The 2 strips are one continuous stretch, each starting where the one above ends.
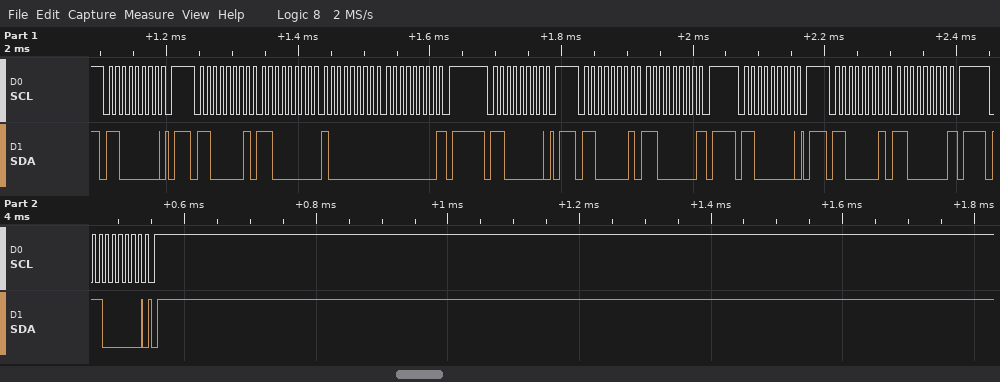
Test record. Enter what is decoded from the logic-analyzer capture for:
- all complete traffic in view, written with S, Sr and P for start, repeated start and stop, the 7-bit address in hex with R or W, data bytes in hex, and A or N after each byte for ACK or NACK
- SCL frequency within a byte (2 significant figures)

S 60W A P S 60R A C0 A 80 A 00 N P S 60W A P S 60R A C0 N P S 60W A P S 60R A C0 N P S 60W A P
100 kHz
